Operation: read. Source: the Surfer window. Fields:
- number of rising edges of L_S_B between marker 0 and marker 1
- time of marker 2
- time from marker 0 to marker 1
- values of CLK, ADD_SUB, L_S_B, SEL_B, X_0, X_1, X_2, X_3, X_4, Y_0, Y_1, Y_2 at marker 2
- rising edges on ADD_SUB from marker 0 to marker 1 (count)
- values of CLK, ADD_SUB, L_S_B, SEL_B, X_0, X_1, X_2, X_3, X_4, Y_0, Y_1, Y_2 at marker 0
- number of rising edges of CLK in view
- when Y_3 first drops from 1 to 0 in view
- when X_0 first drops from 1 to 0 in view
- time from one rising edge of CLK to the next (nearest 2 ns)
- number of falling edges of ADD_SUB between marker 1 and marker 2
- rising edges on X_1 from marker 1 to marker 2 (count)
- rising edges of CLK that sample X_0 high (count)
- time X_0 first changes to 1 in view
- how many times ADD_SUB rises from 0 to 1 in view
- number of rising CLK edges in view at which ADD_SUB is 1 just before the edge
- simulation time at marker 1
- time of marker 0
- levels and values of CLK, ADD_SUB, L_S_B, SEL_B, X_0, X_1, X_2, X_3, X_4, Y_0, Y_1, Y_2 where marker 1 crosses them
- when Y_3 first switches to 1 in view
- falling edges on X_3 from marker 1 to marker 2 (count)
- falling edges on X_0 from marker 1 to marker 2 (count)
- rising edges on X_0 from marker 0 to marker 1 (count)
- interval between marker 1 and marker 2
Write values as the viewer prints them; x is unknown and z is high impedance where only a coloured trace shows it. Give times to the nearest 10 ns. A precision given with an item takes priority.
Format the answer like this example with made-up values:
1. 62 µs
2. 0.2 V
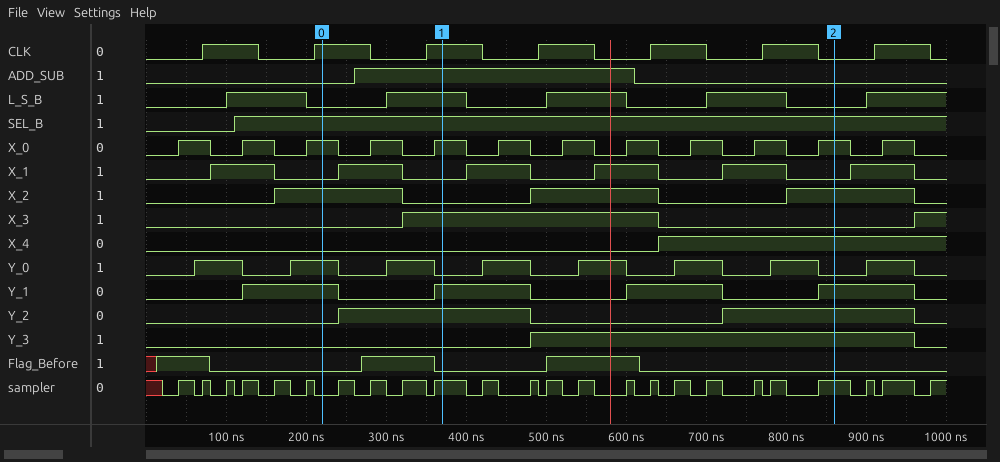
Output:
1. 1
2. 860 ns
3. 150 ns
4. CLK=0, ADD_SUB=0, L_S_B=0, SEL_B=1, X_0=1, X_1=0, X_2=1, X_3=0, X_4=1, Y_0=0, Y_1=1, Y_2=1
5. 1
6. CLK=1, ADD_SUB=0, L_S_B=0, SEL_B=1, X_0=1, X_1=0, X_2=1, X_3=0, X_4=0, Y_0=1, Y_1=1, Y_2=0
7. 7
8. 960 ns
9. 80 ns
10. 140 ns
11. 1
12. 3
13. 4
14. 40 ns
15. 1
16. 2
17. 370 ns
18. 220 ns
19. CLK=1, ADD_SUB=1, L_S_B=1, SEL_B=1, X_0=1, X_1=0, X_2=0, X_3=1, X_4=0, Y_0=0, Y_1=1, Y_2=1
20. 480 ns
21. 1
22. 6
23. 2
24. 490 ns
